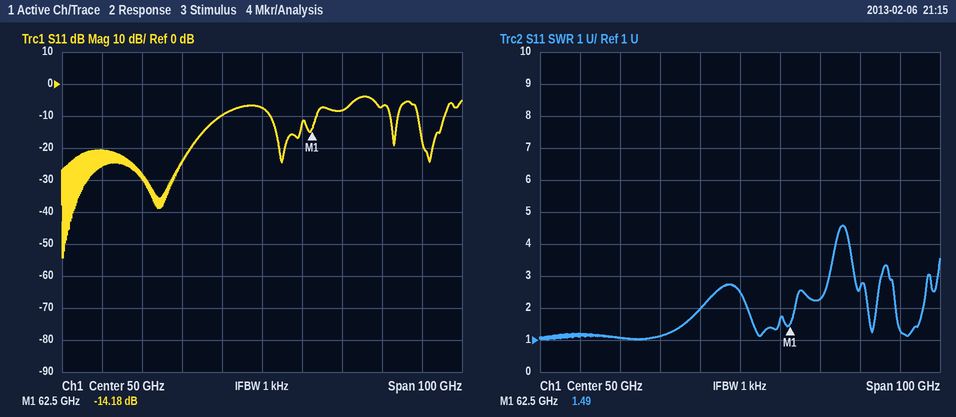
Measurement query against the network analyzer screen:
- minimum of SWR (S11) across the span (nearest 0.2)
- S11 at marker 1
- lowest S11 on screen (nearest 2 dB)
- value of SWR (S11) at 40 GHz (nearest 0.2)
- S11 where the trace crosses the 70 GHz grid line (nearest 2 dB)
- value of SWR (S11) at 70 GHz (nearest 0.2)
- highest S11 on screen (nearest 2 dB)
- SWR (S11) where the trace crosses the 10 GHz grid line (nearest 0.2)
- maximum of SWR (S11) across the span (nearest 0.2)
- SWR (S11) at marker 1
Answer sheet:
1.0
-14.18 dB
-54 dB
2.0
-8 dB
2.2
-4 dB
1.2
4.6
1.49
